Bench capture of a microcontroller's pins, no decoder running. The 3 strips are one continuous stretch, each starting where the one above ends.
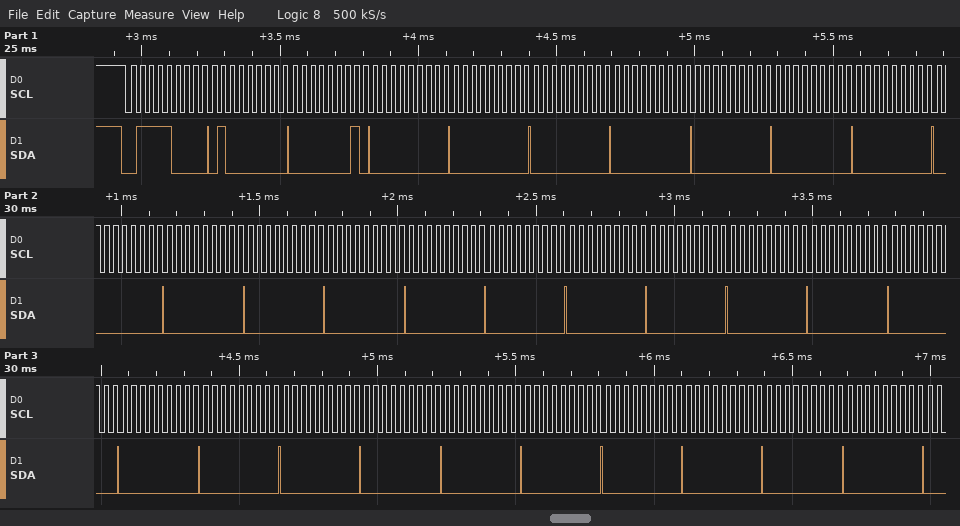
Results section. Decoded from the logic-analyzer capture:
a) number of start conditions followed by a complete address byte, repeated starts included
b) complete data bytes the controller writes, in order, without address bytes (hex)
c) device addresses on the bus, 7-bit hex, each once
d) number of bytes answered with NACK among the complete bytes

1
40 01 00 00 00 00 00 00 00 00 00 00 00 00 00 00 00 00 00 00 00 00 00 00 00 00 00 00 00 00
0x3C
0
